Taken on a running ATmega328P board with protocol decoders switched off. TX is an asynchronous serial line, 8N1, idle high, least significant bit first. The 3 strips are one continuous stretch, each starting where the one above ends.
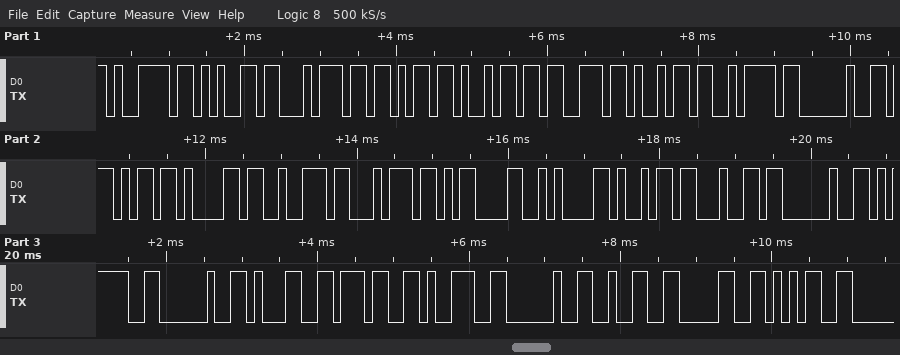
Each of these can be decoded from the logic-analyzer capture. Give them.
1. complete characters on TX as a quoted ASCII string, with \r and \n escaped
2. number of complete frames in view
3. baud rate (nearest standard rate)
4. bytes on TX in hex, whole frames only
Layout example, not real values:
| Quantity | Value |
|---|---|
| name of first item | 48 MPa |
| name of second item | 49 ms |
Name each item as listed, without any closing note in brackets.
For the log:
| Quantity | Value |
|---|---|
| complete characters on TX as a quoted ASCII string, with \r and \n escaped | "yetkisiz kart\r\nid = 179 205" |
| number of complete frames in view | 27 |
| baud rate | 9600 baud |
| bytes on TX in hex, whole frames only | 79 65 74 6B 69 73 69 7A 20 6B 61 72 74 0D 0A 69 64 20 3D 20 31 37 39 20 32 30 35 |
